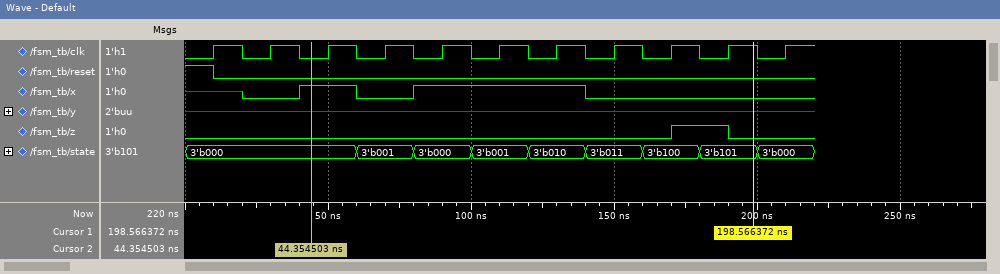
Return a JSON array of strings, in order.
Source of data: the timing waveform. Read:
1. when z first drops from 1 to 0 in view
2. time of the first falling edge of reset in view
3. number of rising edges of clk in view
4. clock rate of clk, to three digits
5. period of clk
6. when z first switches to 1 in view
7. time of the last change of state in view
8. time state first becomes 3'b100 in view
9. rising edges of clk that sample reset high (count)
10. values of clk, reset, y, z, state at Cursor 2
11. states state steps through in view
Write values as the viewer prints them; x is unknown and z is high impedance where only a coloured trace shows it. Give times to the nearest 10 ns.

["190 ns", "10 ns", "11", "50.0 MHz", "20 ns", "170 ns", "200 ns", "160 ns", "1", "clk=0, reset=0, y=x, z=0, state=3'b000", "3'b000, 3'b001, 3'b000, 3'b001, 3'b010, 3'b011, 3'b100, 3'b101, 3'b000"]
